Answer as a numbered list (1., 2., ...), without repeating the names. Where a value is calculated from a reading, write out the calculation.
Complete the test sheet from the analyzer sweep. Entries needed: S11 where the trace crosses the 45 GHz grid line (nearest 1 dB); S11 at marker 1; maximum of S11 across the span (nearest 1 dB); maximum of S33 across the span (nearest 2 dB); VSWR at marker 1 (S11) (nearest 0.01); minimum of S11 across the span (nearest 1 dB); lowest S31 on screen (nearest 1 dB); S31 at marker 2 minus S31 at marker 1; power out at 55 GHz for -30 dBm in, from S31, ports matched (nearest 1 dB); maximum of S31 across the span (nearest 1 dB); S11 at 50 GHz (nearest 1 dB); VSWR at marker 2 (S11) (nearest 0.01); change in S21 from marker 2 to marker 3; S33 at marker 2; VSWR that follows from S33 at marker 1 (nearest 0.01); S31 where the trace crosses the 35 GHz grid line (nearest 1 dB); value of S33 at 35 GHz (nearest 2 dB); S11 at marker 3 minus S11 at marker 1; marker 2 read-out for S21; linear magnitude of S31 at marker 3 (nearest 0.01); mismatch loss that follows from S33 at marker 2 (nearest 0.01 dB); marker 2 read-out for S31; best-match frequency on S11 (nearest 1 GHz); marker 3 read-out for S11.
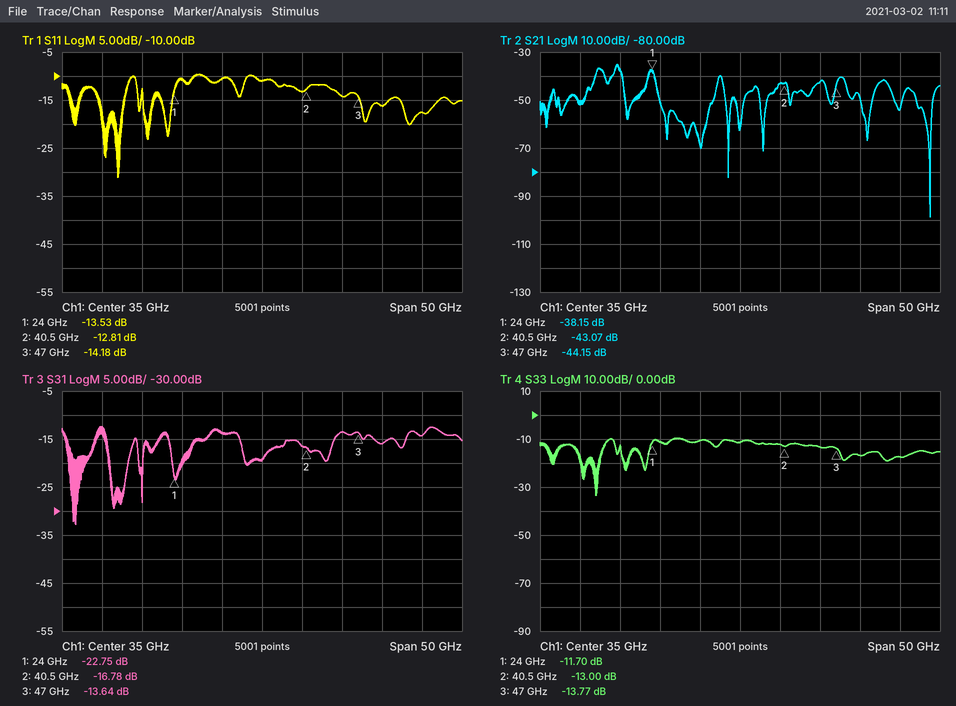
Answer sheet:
1. -14 dB
2. -13.53 dB
3. -10 dB
4. -10 dB
5. (1 + 0.2106)/(1 − 0.2106) ≈ 1.53
6. -31 dB
7. -33 dB
8. -16.78 − (-22.75) = 5.97 dB
9. -30 dBm + (-14 dB) = -44 dBm
10. -12 dB
11. -16 dB
12. (1 + 0.2288)/(1 − 0.2288) ≈ 1.59
13. -44.15 − (-43.07) = -1.08 dB
14. -13.00 dB
15. (1 + 0.2600)/(1 − 0.2600) ≈ 1.70
16. -19 dB
17. -12 dB
18. -14.18 − (-13.53) = -0.65 dB
19. -43.07 dB
20. 10^(-13.64/20) ≈ 0.21
21. −10 log10(1 − 10^(-13/10)) ≈ 0.22 dB
22. -16.78 dB
23. 17 GHz
24. -14.18 dB
